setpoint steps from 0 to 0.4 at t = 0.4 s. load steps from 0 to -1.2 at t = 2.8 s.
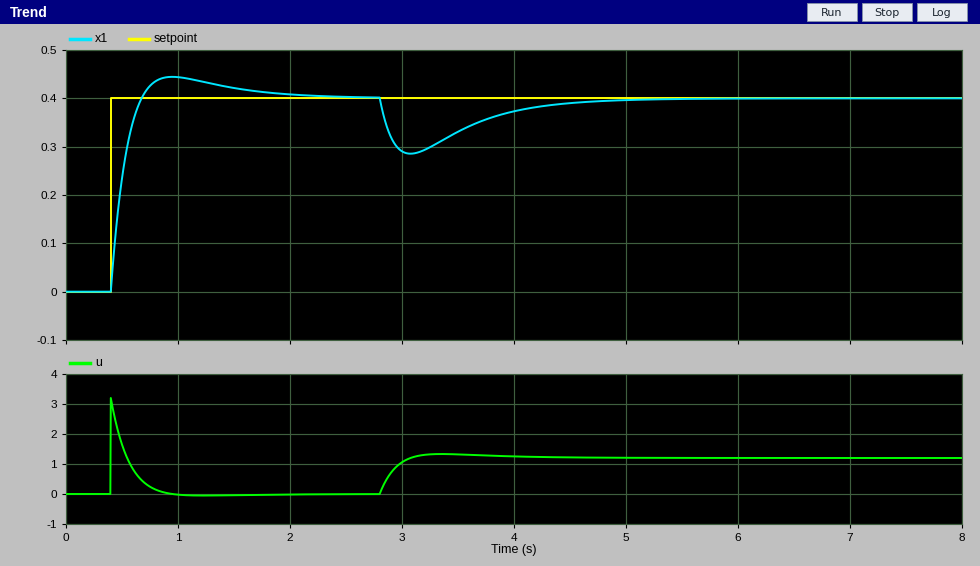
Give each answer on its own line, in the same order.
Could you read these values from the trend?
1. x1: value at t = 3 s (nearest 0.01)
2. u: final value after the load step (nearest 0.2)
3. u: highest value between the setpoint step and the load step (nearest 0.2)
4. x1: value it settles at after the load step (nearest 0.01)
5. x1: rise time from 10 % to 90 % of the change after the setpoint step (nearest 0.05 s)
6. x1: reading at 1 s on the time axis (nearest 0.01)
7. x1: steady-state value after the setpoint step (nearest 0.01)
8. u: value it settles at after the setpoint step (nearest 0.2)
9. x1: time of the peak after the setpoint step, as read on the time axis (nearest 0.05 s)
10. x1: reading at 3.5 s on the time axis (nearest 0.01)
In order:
0.29
1.2
3.2
0.40
0.20 s
0.44
0.40
0.0
0.95 s
0.33
